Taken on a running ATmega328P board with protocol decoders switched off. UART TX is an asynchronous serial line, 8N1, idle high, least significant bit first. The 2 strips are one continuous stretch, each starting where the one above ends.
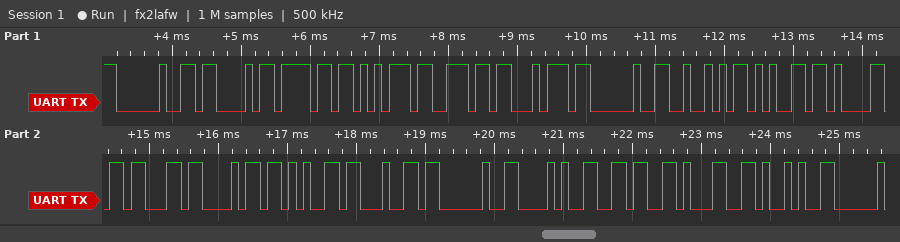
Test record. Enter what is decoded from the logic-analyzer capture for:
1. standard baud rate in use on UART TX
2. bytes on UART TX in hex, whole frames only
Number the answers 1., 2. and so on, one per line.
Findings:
1. 9600 baud
2. 20 43 6F 75 6E 74 20 52 65 61 63 68 65 64 20 28 36 31 29
